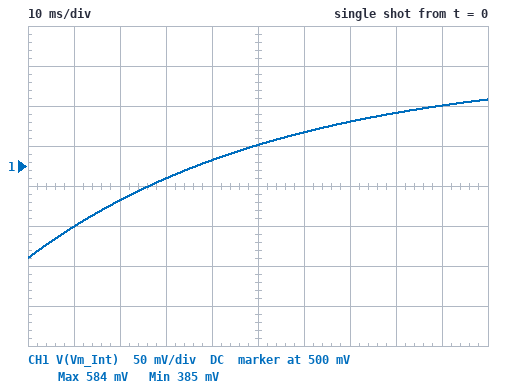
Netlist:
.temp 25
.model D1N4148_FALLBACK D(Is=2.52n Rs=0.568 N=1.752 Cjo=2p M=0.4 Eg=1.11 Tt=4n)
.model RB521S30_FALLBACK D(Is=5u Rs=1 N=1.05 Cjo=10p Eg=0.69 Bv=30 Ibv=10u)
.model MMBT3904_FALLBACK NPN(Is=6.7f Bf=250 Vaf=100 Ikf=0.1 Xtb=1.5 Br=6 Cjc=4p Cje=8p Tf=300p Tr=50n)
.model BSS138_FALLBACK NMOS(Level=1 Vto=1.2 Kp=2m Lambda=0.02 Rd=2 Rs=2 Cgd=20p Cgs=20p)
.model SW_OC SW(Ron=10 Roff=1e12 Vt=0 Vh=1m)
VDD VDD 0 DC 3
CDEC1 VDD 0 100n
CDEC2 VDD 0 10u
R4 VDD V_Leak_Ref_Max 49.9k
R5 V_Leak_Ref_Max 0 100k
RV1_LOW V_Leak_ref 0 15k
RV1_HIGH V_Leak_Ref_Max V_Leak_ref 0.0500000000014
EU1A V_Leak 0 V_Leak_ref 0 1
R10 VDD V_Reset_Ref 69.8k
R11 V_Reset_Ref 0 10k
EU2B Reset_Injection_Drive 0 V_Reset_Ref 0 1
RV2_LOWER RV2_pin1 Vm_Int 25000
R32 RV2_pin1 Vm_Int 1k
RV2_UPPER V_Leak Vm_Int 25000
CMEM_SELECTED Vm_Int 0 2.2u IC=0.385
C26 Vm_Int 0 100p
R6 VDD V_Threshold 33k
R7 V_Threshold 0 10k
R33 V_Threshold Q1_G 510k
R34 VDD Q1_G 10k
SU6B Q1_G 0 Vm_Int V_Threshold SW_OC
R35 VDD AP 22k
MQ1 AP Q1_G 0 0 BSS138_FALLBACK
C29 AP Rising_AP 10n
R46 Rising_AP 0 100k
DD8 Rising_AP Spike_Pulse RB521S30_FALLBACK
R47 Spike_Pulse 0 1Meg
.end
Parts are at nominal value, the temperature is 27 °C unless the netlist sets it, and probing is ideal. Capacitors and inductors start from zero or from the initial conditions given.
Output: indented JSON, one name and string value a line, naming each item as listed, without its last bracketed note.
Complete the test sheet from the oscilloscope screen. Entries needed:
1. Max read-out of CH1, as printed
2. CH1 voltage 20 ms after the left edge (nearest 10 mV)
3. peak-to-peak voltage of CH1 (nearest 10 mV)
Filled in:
{
  "Max read-out of CH1, as printed": "584 mV",
  "CH1 voltage 20 ms after the left edge": "460 mV",
  "peak-to-peak voltage of CH1": "200 mV"
}
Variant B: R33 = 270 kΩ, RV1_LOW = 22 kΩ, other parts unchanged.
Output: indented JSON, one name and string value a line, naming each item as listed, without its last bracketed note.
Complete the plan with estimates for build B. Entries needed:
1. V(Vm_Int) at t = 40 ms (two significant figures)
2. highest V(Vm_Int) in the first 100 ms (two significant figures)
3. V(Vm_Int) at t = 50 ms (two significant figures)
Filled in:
{
  "V(Vm_Int) at t = 40 ms": "600 mV",
  "highest V(Vm_Int) in the first 100 ms": "730 mV",
  "V(Vm_Int) at t = 50 ms": "630 mV"
}
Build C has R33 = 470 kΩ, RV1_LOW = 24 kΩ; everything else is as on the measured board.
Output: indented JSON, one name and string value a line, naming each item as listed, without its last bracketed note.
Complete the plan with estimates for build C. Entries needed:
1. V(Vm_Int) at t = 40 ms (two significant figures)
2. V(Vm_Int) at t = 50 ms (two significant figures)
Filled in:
{
  "V(Vm_Int) at t = 40 ms": "620 mV",
  "V(Vm_Int) at t = 50 ms": "660 mV"
}
